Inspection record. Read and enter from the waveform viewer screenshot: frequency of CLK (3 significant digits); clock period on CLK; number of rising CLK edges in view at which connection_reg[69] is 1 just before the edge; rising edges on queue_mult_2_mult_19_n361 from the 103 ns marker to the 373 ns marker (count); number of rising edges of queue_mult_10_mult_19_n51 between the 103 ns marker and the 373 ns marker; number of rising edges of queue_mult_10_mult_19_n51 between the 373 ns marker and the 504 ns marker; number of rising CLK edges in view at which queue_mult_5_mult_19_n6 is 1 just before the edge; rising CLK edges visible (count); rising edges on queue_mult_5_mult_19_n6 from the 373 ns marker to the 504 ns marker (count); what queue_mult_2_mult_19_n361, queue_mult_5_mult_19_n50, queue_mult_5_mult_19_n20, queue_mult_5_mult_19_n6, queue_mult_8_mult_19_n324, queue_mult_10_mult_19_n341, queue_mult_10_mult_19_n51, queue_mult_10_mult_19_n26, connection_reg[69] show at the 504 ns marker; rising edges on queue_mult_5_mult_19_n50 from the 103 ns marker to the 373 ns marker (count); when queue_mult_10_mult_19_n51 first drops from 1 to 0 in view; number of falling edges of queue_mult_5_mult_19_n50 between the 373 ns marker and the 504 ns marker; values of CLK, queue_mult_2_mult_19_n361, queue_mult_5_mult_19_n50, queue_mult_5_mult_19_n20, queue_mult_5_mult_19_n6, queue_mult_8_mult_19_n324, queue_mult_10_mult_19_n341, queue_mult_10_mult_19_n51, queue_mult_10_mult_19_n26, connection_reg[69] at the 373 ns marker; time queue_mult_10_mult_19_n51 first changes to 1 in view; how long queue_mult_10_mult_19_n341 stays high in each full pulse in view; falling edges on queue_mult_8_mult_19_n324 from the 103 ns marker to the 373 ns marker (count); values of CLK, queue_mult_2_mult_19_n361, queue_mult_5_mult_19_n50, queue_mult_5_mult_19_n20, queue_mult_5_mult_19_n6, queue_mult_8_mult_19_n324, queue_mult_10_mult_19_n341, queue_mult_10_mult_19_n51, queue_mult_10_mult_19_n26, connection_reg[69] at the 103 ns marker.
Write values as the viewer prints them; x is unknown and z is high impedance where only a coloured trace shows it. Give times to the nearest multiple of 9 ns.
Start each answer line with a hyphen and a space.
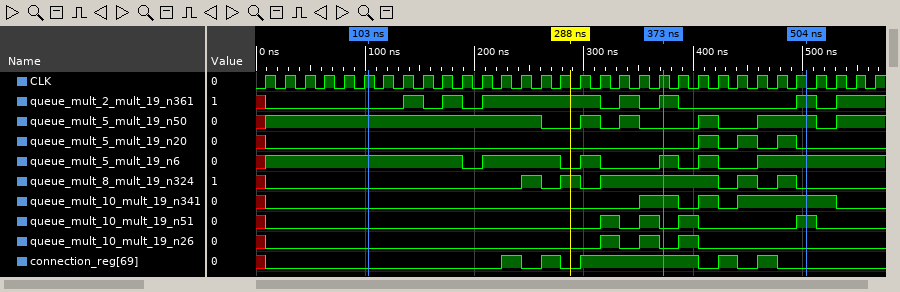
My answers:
- 55.6 MHz
- 18 ns
- 10
- 5
- 2
- 2
- 23
- 32
- 2
- queue_mult_2_mult_19_n361=1, queue_mult_5_mult_19_n50=1, queue_mult_5_mult_19_n20=0, queue_mult_5_mult_19_n6=1, queue_mult_8_mult_19_n324=0, queue_mult_10_mult_19_n341=1, queue_mult_10_mult_19_n51=1, queue_mult_10_mult_19_n26=0, connection_reg[69]=0
- 2
- 333 ns
- 1
- CLK=1, queue_mult_2_mult_19_n361=1, queue_mult_5_mult_19_n50=0, queue_mult_5_mult_19_n20=0, queue_mult_5_mult_19_n6=1, queue_mult_8_mult_19_n324=1, queue_mult_10_mult_19_n341=1, queue_mult_10_mult_19_n51=0, queue_mult_10_mult_19_n26=0, connection_reg[69]=1
- 315 ns
- 36 ns, 18 ns, 90 ns
- 2
- CLK=1, queue_mult_2_mult_19_n361=0, queue_mult_5_mult_19_n50=1, queue_mult_5_mult_19_n20=0, queue_mult_5_mult_19_n6=1, queue_mult_8_mult_19_n324=0, queue_mult_10_mult_19_n341=0, queue_mult_10_mult_19_n51=0, queue_mult_10_mult_19_n26=0, connection_reg[69]=0
